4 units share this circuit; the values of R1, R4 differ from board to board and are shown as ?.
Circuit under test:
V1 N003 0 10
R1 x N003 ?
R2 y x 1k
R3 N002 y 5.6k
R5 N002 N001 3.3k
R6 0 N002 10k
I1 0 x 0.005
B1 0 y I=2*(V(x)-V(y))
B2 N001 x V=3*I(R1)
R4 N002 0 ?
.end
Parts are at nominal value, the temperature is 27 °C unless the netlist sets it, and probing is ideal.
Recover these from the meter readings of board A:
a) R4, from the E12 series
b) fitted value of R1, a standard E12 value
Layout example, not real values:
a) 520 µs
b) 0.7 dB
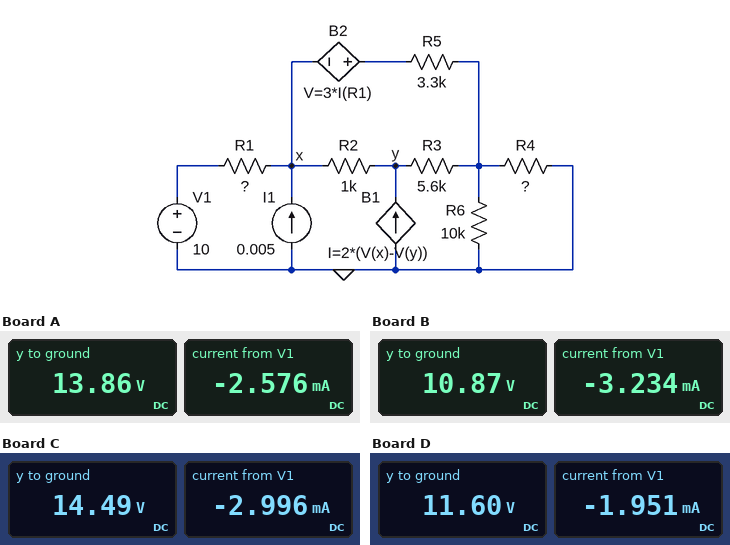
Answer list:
a) 1.8 kΩ
b) 1.5 kΩ
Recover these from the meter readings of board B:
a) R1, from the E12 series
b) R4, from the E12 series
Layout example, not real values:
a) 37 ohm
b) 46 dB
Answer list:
a) 270 Ω
b) 2.2 kΩ
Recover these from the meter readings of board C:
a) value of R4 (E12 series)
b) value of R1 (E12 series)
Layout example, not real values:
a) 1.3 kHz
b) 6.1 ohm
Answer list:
a) 3.3 kΩ
b) 1.5 kΩ
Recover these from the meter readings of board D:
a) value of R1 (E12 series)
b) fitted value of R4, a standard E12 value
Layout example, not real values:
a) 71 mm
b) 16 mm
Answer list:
a) 820 Ω
b) 330 Ω
